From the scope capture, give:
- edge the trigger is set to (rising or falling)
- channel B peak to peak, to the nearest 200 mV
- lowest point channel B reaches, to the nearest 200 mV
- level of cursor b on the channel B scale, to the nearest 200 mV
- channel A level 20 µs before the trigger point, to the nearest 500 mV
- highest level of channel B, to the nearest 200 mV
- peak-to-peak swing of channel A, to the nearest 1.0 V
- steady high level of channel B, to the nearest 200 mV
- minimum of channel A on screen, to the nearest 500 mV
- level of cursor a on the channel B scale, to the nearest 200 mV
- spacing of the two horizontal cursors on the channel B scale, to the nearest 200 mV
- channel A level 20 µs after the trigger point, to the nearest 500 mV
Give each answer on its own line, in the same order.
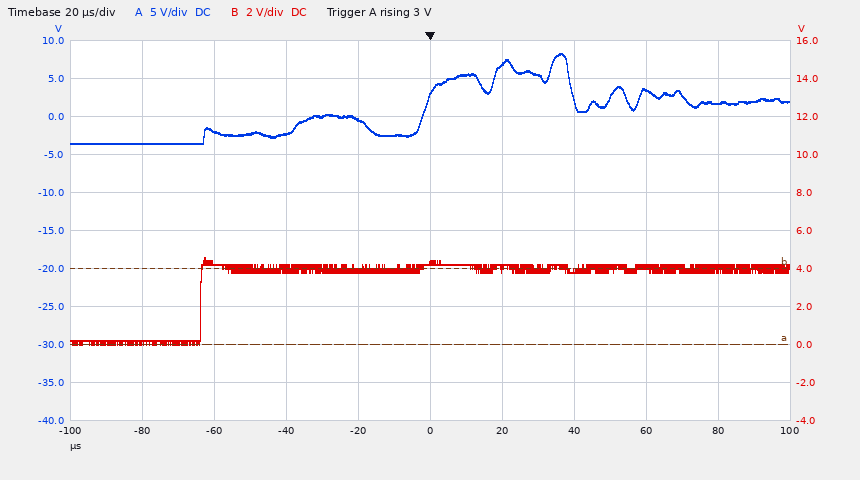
rising
4.6 V
0.0 V
4.0 V
-500 mV
4.6 V
12.0 V
4.0 V
-3.5 V
0.0 V
4.0 V
7.0 V
